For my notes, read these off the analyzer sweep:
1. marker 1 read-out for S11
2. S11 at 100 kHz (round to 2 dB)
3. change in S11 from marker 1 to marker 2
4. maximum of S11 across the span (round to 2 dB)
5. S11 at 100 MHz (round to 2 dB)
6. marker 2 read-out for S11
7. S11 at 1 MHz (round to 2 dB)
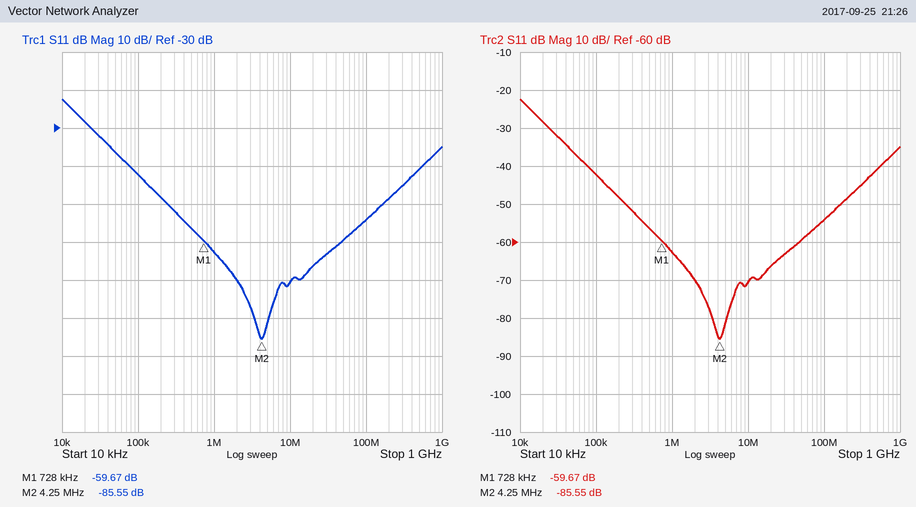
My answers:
-59.67 dB
-42 dB
-25.88 dB
-22 dB
-54 dB
-85.55 dB
-62 dB
